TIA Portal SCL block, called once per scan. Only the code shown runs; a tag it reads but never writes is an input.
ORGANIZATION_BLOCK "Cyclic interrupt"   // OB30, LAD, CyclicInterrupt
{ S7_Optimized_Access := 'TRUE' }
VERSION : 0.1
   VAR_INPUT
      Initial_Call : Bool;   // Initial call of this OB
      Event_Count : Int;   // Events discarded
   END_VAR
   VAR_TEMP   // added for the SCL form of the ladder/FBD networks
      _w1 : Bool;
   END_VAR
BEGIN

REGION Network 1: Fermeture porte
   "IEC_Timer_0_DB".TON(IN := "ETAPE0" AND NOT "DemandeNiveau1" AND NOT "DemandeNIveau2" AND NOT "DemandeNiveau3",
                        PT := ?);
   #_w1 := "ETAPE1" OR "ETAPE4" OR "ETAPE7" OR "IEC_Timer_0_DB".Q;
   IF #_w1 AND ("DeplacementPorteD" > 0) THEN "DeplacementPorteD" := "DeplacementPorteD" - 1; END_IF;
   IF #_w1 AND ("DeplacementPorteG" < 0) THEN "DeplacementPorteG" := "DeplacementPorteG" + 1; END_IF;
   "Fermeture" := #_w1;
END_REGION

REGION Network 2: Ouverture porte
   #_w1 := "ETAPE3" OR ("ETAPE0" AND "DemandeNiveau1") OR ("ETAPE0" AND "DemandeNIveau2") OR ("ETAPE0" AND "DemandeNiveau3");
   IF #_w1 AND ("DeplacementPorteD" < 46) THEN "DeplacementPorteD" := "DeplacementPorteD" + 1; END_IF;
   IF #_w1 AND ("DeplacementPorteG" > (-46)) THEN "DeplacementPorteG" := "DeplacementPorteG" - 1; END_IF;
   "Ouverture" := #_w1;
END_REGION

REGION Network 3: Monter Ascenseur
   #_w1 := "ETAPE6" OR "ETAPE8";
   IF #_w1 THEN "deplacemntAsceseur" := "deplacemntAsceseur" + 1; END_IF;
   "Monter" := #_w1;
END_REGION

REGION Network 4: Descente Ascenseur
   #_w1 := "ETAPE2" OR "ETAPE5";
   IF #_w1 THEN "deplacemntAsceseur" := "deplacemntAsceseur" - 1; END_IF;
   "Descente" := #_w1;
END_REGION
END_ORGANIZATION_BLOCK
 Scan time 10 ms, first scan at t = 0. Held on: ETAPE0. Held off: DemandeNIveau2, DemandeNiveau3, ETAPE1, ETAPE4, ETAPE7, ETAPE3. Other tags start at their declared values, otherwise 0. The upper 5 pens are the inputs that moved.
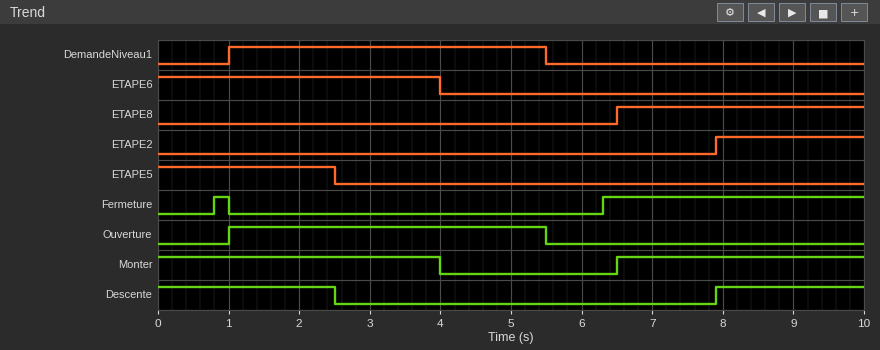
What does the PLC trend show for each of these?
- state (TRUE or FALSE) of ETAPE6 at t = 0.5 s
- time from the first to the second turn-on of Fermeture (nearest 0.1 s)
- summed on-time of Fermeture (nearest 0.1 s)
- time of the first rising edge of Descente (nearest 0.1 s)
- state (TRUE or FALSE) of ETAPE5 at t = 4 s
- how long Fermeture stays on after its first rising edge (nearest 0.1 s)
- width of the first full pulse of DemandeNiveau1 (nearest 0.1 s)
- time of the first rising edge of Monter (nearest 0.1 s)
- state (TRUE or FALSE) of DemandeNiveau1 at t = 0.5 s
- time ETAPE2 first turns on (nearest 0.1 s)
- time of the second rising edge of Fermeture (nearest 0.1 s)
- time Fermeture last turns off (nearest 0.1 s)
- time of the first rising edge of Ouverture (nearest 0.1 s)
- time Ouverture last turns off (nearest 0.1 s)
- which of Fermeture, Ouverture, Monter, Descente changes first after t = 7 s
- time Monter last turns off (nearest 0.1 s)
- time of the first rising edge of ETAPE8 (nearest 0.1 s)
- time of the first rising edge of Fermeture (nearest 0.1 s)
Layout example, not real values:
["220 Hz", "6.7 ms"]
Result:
["TRUE", "5.5 s", "3.9 s", "7.9 s", "FALSE", "0.2 s", "4.5 s", "6.5 s", "FALSE", "7.9 s", "6.3 s", "1.0 s", "1.0 s", "5.5 s", "Descente", "4.0 s", "6.5 s", "0.8 s"]
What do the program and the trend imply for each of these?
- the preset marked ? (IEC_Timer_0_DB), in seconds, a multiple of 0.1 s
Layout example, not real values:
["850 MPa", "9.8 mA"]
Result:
["0.8 s"]
